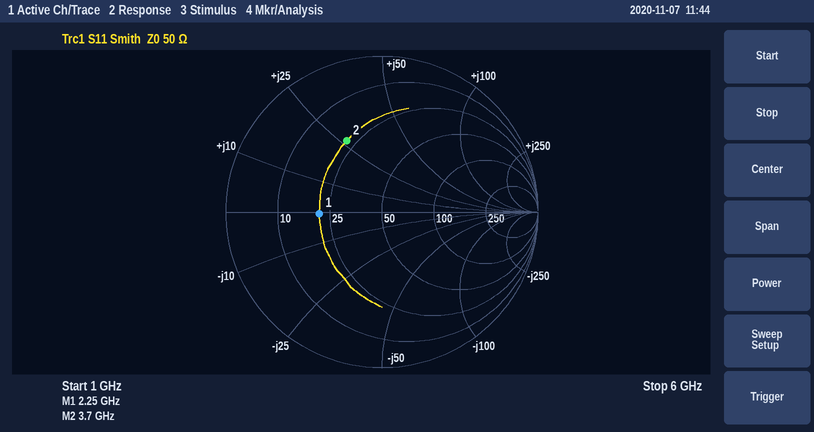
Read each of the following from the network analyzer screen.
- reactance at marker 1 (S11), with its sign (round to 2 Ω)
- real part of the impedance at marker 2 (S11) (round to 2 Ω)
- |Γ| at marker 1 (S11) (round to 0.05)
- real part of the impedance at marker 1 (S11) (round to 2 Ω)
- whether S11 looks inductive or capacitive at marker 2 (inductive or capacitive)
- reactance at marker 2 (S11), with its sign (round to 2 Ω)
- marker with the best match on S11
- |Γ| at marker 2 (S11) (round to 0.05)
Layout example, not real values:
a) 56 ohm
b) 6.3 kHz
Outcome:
a) 0 Ω
b) 22 Ω
c) 0.40
d) 22 Ω
e) inductive
f) +26 Ω
g) marker 1
h) 0.50
